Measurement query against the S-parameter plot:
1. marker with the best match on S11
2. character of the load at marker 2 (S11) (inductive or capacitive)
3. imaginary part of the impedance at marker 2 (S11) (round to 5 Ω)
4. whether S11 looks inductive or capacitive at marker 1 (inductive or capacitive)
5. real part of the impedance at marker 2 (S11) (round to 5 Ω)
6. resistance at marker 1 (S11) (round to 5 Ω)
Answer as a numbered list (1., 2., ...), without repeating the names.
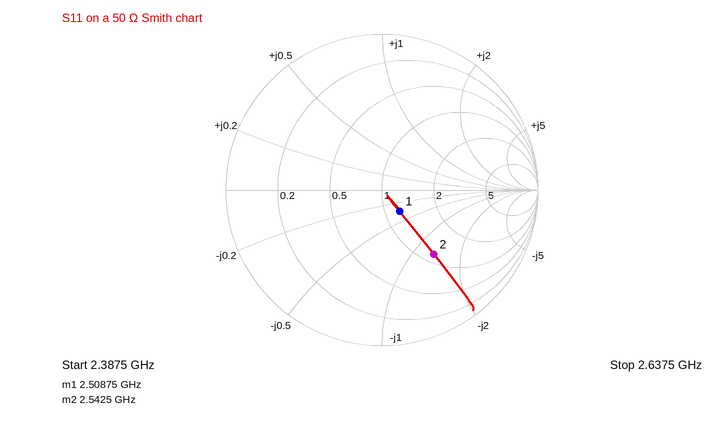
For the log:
1. marker 1
2. capacitive
3. -65 Ω
4. capacitive
5. 60 Ω
6. 60 Ω
